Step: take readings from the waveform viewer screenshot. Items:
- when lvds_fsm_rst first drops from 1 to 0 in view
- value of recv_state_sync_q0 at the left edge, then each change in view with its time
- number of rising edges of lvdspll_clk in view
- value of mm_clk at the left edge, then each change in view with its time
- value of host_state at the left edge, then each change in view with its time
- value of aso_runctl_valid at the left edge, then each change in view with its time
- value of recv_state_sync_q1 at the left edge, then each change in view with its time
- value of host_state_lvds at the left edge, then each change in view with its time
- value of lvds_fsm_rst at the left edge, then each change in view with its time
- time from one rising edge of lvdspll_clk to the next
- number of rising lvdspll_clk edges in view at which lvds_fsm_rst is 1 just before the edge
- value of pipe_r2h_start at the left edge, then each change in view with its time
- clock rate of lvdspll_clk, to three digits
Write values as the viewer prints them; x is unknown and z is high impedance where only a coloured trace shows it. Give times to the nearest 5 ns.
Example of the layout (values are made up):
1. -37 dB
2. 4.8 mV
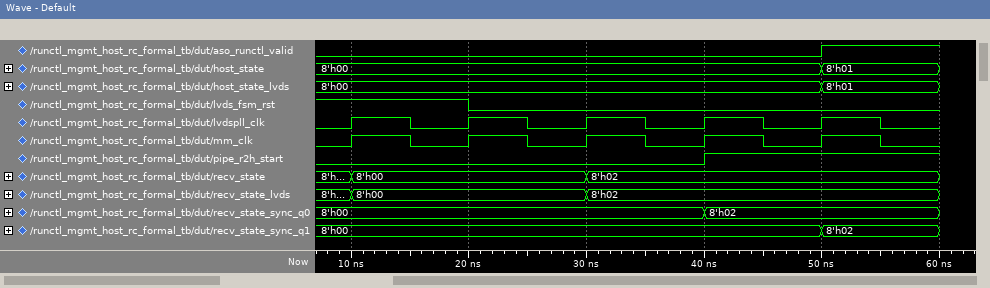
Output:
1. 20 ns
2. 8'h00, 8'h02 at 40 ns
3. 5
4. 0, 1 at 10 ns, 0 at 15 ns, 1 at 20 ns, 0 at 25 ns, 1 at 30 ns, 0 at 35 ns, 1 at 40 ns, 0 at 45 ns, 1 at 50 ns, 0 at 55 ns
5. 8'h00, 8'h01 at 50 ns
6. 0, 1 at 50 ns
7. 8'h00, 8'h02 at 50 ns
8. 8'h00, 8'h01 at 50 ns
9. 1, 0 at 20 ns
10. 10 ns
11. 2
12. 0, 1 at 40 ns
13. 100 MHz
